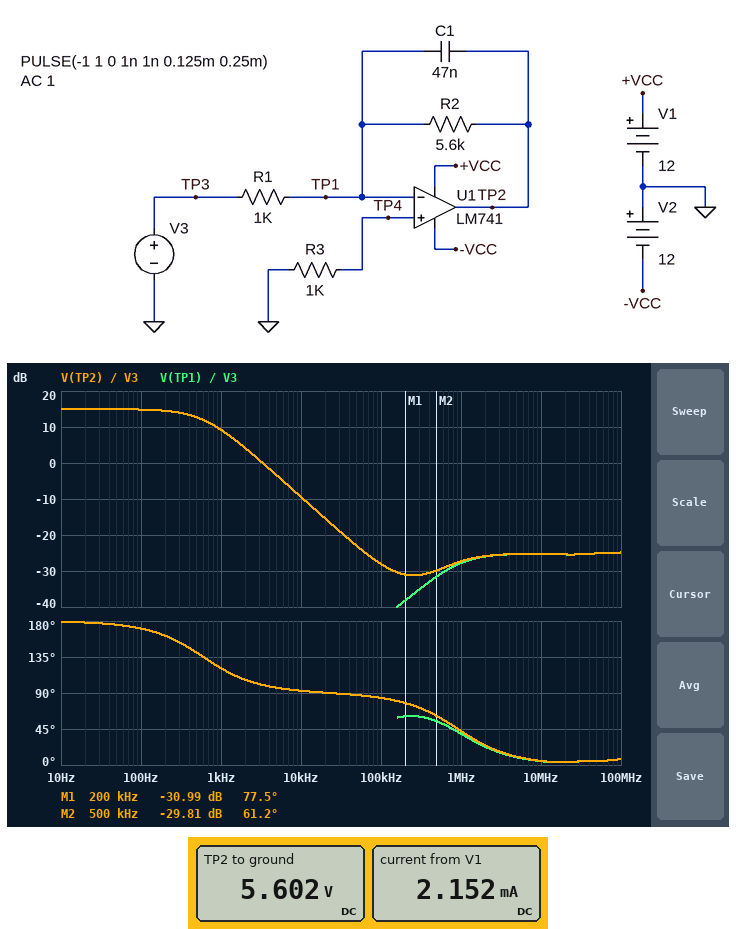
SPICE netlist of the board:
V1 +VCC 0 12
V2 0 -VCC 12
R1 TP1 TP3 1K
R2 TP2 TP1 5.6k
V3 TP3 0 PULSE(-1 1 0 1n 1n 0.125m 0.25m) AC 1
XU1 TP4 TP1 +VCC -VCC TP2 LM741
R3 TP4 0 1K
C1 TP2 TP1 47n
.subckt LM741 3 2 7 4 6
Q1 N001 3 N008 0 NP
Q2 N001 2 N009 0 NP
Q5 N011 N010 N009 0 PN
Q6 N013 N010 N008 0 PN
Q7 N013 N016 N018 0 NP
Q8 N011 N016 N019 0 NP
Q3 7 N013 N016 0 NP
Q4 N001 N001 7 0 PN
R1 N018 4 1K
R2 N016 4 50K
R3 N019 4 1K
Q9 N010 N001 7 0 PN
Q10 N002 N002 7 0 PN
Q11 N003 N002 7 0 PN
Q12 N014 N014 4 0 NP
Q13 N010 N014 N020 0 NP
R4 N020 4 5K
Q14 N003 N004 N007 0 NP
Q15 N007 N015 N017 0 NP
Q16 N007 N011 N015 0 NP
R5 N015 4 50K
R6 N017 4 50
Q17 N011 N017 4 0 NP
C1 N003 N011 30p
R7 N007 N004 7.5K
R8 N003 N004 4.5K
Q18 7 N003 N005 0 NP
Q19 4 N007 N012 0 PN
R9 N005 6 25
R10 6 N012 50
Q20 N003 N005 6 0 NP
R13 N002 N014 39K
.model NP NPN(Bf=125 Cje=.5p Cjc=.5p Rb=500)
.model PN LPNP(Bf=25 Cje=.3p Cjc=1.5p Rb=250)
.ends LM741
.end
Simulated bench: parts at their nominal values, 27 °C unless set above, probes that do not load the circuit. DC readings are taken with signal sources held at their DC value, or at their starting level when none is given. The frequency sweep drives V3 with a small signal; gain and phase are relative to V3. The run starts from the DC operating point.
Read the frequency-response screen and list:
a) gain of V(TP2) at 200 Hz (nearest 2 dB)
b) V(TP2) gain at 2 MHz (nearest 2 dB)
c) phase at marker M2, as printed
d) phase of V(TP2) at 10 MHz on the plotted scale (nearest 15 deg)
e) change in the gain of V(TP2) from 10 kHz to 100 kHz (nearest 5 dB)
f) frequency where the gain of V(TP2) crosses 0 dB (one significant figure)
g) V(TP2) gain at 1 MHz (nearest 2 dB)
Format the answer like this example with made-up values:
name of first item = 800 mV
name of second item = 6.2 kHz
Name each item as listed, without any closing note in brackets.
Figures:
gain of V(TP2) at 200 Hz = 14 dB
V(TP2) gain at 2 MHz = -26 dB
phase at marker M2, as printed = 61.2 deg
phase of V(TP2) at 10 MHz on the plotted scale = 0 deg
change in the gain of V(TP2) from 10 kHz to 100 kHz = -20 dB
frequency where the gain of V(TP2) crosses 0 dB = 3 kHz
V(TP2) gain at 1 MHz = -28 dB
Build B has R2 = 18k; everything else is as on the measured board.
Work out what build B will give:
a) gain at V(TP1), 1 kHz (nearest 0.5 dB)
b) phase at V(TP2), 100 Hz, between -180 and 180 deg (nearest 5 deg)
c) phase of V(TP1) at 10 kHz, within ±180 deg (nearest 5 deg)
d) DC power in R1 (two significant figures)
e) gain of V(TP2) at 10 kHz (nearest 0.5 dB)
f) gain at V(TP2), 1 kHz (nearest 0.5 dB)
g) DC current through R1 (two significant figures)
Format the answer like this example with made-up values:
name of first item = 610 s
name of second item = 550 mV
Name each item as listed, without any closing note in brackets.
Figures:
gain at V(TP1), 1 kHz = -1.0 dB
phase at V(TP2), 100 Hz, between -180 and 180 deg = 25 deg
phase of V(TP1) at 10 kHz, within ±180 deg = -60 deg
DC power in R1 = 410 µW
gain of V(TP2) at 10 kHz = -24.0 dB
gain at V(TP2), 1 kHz = -34.5 dB
DC current through R1 = 640 µA
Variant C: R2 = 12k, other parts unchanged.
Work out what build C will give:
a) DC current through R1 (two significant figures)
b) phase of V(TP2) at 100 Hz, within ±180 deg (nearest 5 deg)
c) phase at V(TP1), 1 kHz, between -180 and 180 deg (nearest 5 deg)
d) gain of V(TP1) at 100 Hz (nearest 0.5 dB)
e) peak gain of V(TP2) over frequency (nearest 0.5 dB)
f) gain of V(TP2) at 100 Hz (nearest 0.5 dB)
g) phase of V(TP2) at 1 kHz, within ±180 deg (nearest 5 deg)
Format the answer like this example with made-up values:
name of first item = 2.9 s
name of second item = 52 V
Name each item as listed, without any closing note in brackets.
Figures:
DC current through R1 = 940 µA
phase of V(TP2) at 100 Hz, within ±180 deg = 20 deg
phase at V(TP1), 1 kHz, between -180 and 180 deg = -15 deg
gain of V(TP1) at 100 Hz = -0.5 dB
peak gain of V(TP2) over frequency = -22.0 dB
gain of V(TP2) at 100 Hz = -46.5 dB
phase of V(TP2) at 1 kHz, within ±180 deg = 60 deg
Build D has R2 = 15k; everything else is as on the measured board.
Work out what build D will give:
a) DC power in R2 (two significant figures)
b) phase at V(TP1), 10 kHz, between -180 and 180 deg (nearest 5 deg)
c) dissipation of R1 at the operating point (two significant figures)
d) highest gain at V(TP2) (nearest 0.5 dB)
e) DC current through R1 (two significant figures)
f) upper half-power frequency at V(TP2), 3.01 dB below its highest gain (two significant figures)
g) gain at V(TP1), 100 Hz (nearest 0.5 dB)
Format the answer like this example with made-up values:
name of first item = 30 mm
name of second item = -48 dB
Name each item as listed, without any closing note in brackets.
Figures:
DC power in R2 = 8.7 mW
phase at V(TP1), 10 kHz, between -180 and 180 deg = -60 deg
dissipation of R1 at the operating point = 580 µW
highest gain at V(TP2) = -21.0 dB
DC current through R1 = 760 µA
upper half-power frequency at V(TP2), 3.01 dB below its highest gain = 3.1 GHz
gain at V(TP1), 100 Hz = -0.5 dB
